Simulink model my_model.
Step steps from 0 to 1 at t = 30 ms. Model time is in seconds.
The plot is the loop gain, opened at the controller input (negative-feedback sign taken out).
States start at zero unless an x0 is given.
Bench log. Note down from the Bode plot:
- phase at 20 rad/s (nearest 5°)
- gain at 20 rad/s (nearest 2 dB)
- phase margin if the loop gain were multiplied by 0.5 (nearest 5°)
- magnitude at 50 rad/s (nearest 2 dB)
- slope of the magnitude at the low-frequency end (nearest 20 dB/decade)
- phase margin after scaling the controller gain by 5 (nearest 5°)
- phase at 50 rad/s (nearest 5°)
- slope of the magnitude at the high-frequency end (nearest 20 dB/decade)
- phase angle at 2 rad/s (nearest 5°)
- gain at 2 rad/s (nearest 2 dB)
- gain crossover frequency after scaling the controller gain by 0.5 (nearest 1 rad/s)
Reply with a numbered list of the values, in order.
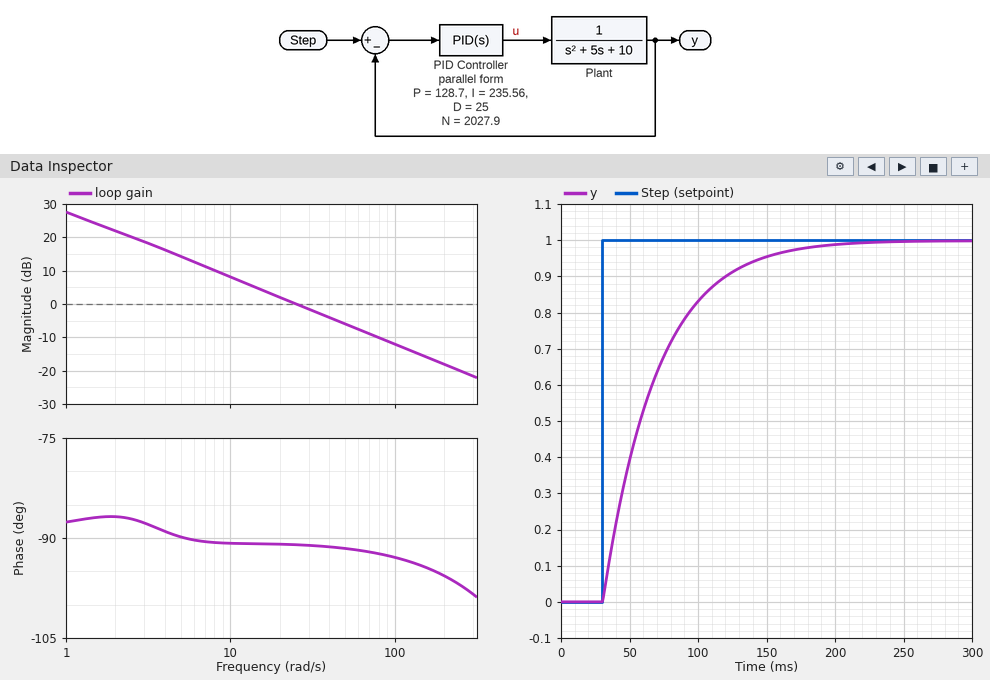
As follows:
1. -90°
2. 2 dB
3. 90°
4. -6 dB
5. -20 dB/decade
6. 85°
7. -90°
8. -20 dB/decade
9. -85°
10. 22 dB
11. 13 rad/s
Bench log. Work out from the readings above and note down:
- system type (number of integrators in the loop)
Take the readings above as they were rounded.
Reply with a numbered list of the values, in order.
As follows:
1. 1
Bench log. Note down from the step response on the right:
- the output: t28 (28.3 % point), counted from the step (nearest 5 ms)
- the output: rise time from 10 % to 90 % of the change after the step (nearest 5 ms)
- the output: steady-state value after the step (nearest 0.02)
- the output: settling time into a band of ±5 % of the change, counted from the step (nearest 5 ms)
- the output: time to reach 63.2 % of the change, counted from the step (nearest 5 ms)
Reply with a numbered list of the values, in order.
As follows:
1. 15 ms
2. 85 ms
3. 1.00
4. 115 ms
5. 40 ms
